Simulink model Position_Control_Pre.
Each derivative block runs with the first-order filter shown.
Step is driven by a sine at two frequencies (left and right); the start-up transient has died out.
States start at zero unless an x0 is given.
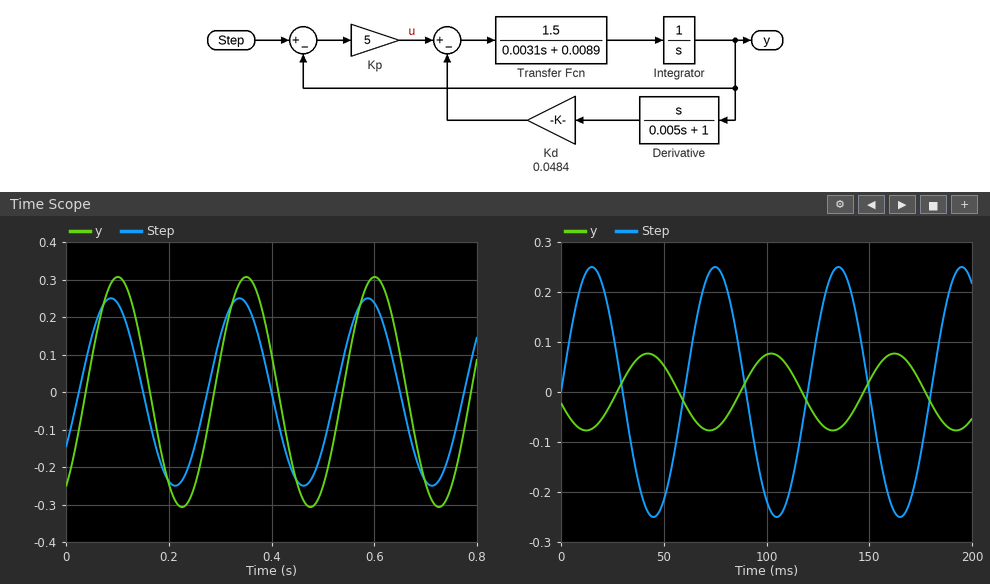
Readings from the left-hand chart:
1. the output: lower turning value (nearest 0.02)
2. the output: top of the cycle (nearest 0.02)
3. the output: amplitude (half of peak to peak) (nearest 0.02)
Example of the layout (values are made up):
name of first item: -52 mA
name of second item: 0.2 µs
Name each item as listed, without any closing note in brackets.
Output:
the output: lower turning value: -0.30
the output: top of the cycle: 0.30
the output: amplitude (half of peak to peak): 0.30
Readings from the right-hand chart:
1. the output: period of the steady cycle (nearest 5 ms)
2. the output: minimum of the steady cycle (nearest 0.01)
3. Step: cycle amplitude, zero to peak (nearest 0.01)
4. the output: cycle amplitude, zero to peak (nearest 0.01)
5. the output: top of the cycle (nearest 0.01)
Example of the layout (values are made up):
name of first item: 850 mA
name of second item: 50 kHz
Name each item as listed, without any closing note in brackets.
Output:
the output: period of the steady cycle: 60 ms
the output: minimum of the steady cycle: -0.08
Step: cycle amplitude, zero to peak: 0.25
the output: cycle amplitude, zero to peak: 0.08
the output: top of the cycle: 0.08
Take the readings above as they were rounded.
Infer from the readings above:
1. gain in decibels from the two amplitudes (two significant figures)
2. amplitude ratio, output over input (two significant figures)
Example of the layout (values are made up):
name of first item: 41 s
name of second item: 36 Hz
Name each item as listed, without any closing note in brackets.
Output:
gain in decibels from the two amplitudes: -9.9 dB
amplitude ratio, output over input: 0.32
